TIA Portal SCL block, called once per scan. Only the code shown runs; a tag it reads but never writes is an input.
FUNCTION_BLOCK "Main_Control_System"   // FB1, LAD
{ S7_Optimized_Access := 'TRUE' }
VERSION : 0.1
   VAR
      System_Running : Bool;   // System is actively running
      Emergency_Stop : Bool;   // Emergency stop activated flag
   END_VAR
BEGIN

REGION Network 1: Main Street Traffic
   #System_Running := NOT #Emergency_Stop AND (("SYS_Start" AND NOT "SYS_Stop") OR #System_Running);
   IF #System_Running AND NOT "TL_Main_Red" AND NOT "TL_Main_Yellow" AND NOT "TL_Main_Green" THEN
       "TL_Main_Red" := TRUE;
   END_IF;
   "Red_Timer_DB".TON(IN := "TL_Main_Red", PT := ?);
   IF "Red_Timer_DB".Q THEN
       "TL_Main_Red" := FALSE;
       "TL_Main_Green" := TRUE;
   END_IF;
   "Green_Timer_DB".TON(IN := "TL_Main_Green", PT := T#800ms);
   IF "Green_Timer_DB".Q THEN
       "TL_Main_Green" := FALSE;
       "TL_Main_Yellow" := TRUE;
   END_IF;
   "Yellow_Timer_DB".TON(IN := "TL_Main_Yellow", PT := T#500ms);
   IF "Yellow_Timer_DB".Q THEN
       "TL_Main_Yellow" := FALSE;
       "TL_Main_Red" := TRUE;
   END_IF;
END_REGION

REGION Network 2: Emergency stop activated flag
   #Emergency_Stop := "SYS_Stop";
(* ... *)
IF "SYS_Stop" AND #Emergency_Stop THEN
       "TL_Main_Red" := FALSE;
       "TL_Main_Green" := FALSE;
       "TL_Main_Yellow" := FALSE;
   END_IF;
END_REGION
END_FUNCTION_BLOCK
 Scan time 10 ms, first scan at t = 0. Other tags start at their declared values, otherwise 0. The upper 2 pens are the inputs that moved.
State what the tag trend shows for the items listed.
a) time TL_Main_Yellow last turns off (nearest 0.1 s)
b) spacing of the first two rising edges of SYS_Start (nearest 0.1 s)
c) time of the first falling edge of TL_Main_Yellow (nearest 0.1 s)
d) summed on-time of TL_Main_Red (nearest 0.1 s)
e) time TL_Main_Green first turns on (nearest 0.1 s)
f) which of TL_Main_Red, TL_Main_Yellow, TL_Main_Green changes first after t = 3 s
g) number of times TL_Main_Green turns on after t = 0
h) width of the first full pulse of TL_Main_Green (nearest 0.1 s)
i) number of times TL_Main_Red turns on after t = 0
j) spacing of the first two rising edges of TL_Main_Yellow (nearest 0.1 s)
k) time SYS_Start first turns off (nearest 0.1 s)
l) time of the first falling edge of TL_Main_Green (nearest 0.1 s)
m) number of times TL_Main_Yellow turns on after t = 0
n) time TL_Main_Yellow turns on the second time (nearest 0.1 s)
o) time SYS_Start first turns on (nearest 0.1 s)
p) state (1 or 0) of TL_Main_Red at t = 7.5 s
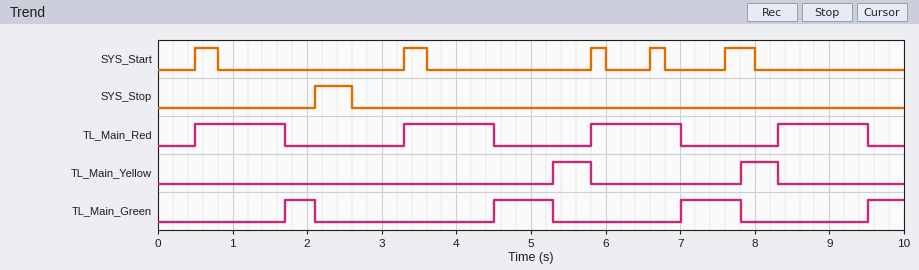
8.3 s
2.8 s
5.8 s
4.8 s
1.7 s
TL_Main_Red
4
0.4 s
4
2.5 s
0.8 s
2.1 s
2
7.8 s
0.5 s
0
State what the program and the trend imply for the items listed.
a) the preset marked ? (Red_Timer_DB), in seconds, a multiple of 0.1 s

1.2 s
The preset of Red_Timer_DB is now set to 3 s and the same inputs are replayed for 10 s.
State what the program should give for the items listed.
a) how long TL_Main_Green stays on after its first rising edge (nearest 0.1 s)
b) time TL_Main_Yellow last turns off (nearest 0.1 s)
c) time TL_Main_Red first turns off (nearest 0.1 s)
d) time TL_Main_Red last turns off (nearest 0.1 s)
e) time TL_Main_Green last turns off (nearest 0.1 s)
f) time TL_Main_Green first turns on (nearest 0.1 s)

0.8 s
7.6 s
2.1 s
6.3 s
7.1 s
6.3 s
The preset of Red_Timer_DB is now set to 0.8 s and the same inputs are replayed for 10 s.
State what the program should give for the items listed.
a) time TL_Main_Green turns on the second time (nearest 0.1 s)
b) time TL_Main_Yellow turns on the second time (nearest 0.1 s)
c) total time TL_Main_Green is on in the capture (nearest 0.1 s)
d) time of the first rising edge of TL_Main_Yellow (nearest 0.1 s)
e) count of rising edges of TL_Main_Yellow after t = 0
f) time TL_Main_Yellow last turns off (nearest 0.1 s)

4.1 s
7.0 s
3.2 s
4.9 s
3
9.6 s
